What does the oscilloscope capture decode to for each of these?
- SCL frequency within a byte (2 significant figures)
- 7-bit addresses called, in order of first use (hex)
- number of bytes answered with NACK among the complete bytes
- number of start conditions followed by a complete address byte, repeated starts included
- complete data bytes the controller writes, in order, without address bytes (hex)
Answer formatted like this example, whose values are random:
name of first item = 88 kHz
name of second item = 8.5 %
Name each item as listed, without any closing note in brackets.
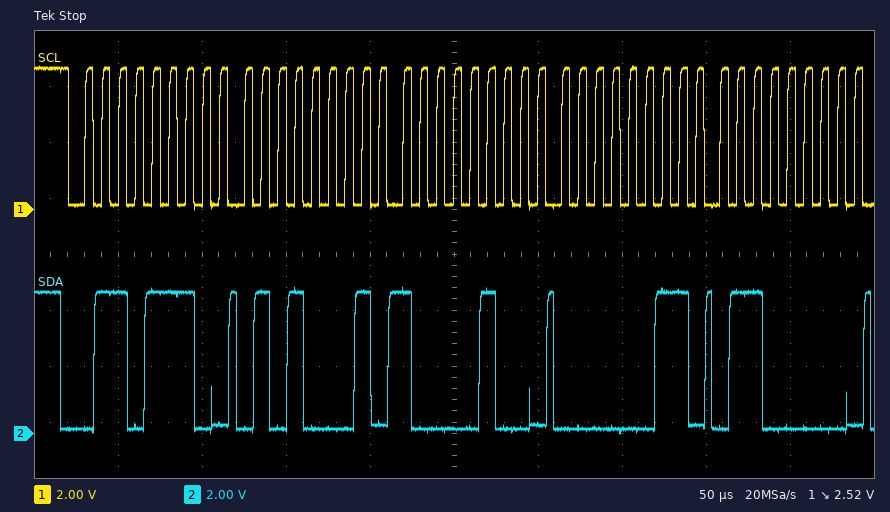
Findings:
SCL frequency within a byte = 100 kHz
7-bit addresses called, in order of first use = 0x37
number of bytes answered with NACK among the complete bytes = 0
number of start conditions followed by a complete address byte, repeated starts included = 1
complete data bytes the controller writes, in order, without address bytes = 51 84 03 60
